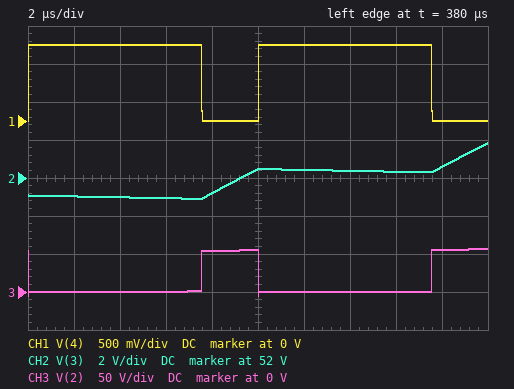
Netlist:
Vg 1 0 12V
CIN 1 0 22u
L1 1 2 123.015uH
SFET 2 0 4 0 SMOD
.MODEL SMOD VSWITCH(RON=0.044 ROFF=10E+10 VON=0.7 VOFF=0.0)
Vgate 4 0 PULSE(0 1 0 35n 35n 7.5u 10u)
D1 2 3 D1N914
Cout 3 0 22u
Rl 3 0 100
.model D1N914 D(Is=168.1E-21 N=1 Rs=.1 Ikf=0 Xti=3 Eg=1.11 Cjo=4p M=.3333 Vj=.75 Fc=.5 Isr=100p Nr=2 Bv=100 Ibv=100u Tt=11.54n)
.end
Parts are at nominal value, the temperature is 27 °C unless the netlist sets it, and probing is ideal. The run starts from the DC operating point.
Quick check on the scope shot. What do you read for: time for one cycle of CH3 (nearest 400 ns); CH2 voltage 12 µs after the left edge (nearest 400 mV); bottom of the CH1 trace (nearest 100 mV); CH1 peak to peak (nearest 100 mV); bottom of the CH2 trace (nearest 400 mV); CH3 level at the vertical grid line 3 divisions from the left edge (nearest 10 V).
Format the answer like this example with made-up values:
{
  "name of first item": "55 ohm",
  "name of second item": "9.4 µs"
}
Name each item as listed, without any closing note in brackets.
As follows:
{
  "time for one cycle of CH3": "10.0 µs",
  "CH2 voltage 12 µs after the left edge": "52.4 V",
  "bottom of the CH1 trace": "0 V",
  "CH1 peak to peak": "1.0 V",
  "bottom of the CH2 trace": "50.8 V",
  "CH3 level at the vertical grid line 3 divisions from the left edge": "0 V"
}
